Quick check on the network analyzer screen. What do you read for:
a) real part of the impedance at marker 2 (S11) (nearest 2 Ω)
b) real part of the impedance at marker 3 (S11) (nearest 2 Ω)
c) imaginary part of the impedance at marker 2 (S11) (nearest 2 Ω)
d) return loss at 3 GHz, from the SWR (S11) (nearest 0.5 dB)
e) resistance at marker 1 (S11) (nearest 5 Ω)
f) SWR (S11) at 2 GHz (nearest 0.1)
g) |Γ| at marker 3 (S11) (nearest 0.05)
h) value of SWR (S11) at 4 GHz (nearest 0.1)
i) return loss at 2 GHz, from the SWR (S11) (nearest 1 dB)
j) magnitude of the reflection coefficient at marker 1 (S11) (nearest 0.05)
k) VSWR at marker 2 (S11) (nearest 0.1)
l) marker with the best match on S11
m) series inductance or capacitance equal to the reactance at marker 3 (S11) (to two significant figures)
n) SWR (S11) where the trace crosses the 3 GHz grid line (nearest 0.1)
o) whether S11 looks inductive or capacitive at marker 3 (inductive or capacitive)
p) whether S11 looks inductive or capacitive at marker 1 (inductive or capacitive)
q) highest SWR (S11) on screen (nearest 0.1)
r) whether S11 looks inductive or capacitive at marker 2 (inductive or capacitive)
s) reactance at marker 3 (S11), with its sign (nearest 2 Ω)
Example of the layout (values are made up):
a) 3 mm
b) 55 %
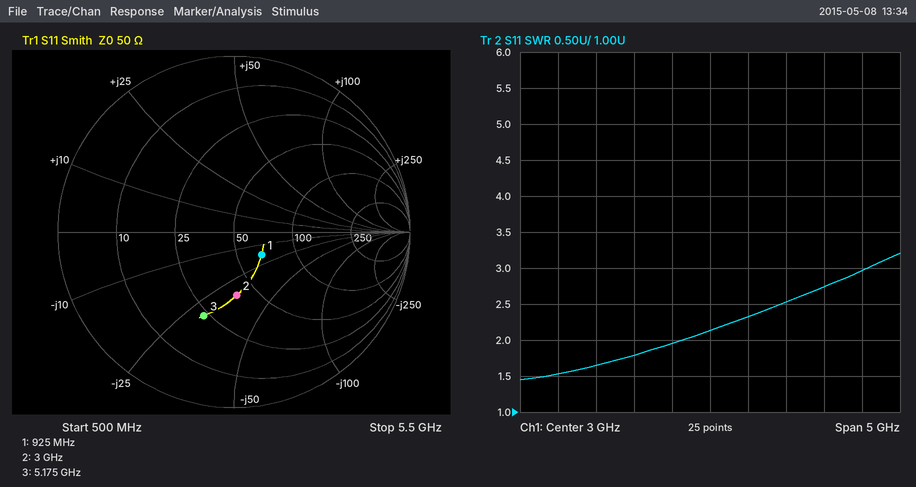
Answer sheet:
a) 40 Ω
b) 24 Ω
c) -32 Ω
d) 9.0 dB
e) 65 Ω
f) 1.8
g) 0.50
h) 2.5
i) 11 dB
j) 0.20
k) 2.1
l) marker 1
m) 1.0 pF
n) 2.1
o) capacitive
p) capacitive
q) 3.2
r) capacitive
s) -30 Ω
